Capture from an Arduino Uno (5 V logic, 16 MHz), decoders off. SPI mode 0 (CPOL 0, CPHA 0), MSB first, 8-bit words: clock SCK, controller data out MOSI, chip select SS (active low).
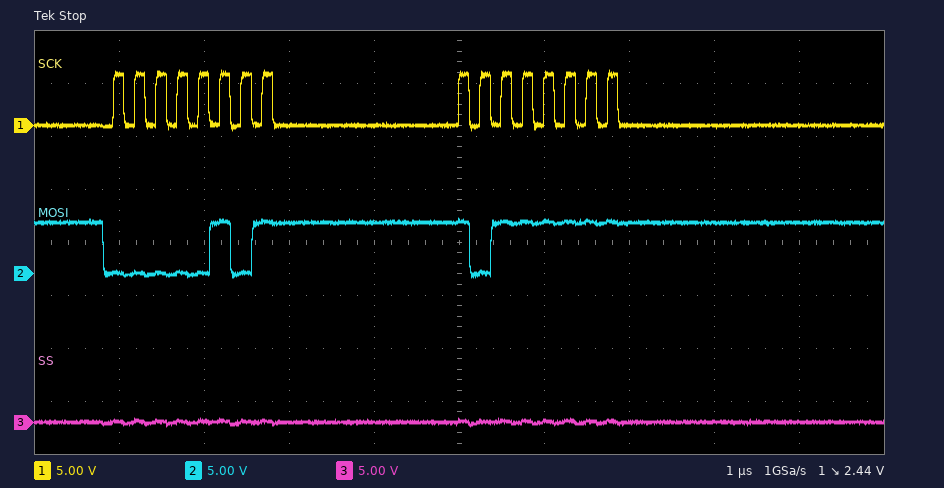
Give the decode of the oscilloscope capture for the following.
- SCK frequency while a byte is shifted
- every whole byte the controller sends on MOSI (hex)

4 MHz
05 BF
